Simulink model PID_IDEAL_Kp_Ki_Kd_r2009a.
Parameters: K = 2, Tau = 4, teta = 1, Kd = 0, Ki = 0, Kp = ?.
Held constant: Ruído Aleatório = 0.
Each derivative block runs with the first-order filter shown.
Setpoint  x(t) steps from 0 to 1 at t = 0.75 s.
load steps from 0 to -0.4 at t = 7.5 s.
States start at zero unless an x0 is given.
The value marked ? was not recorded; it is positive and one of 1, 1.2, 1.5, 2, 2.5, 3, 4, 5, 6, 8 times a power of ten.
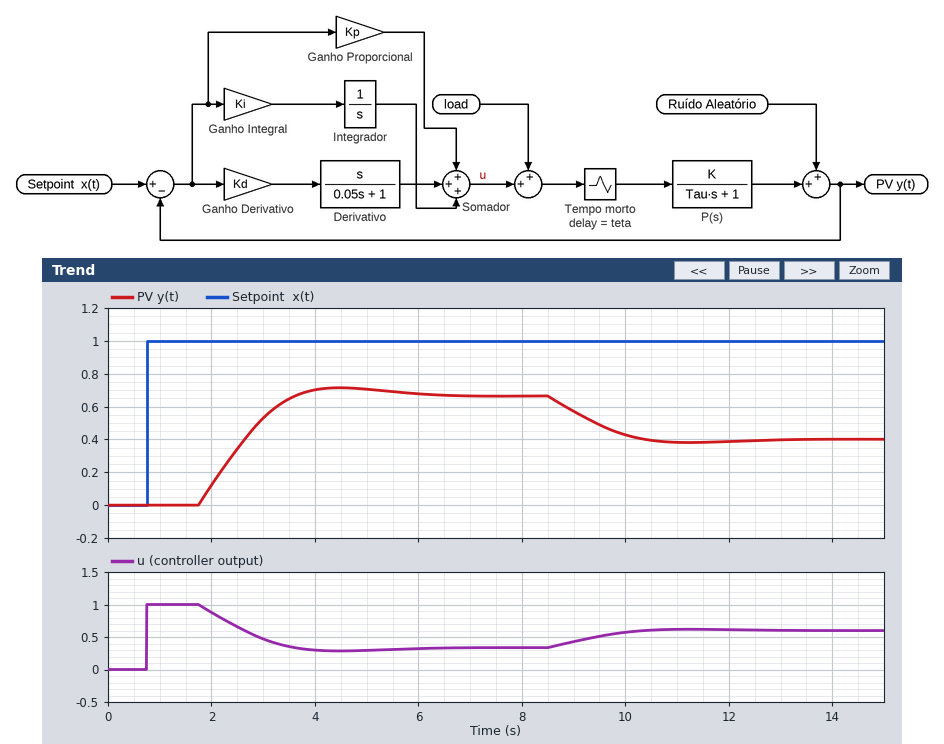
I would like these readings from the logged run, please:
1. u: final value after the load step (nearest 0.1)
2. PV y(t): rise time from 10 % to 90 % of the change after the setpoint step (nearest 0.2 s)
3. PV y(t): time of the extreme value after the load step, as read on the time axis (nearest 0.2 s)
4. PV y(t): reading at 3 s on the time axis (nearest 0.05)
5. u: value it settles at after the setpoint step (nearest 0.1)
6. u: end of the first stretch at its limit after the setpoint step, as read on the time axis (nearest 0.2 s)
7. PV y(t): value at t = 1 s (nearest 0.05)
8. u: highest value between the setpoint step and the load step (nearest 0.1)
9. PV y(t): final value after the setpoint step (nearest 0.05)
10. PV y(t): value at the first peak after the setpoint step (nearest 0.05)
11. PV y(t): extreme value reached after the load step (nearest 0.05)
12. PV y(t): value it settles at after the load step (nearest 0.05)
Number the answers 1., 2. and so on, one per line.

1. 0.6
2. 1.4 s
3. 11.2 s
4. 0.55
5. 0.3
6. 1.8 s
7. 0.00
8. 1.0
9. 0.65
10. 0.70
11. 0.40
12. 0.40
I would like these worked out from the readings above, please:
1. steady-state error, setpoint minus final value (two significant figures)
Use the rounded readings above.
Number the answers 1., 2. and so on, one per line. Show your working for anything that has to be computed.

1. 1 - 0.65 = 0.35
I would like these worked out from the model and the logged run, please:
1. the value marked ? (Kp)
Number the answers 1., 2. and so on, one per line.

1. 1
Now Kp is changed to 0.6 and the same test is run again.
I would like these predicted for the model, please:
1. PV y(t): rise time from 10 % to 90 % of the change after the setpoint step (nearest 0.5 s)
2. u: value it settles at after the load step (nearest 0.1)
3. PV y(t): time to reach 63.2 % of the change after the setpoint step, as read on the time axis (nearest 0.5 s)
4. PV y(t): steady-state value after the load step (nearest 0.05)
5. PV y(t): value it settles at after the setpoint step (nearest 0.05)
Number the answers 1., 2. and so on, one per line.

1. 2.5 s
2. 0.5
3. 3.0 s
4. 0.20
5. 0.55
